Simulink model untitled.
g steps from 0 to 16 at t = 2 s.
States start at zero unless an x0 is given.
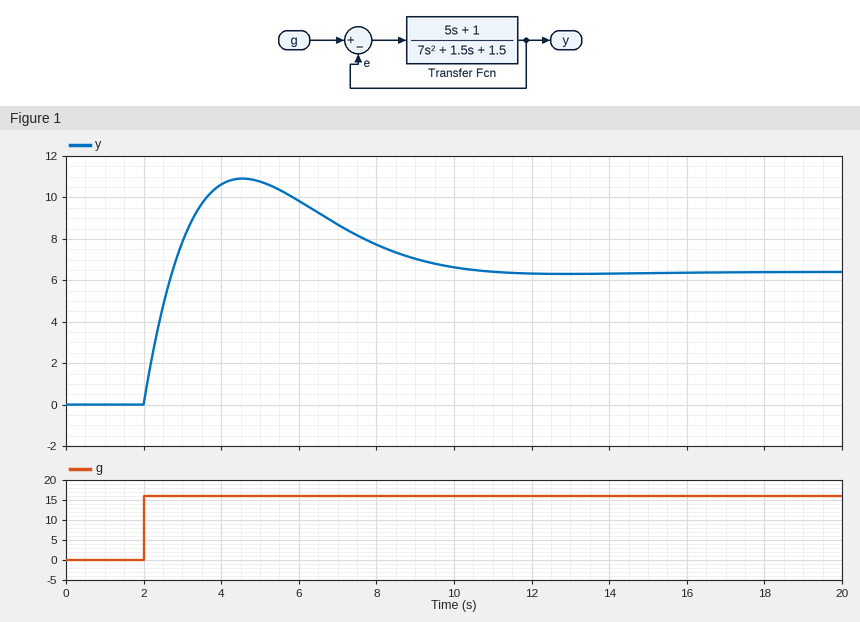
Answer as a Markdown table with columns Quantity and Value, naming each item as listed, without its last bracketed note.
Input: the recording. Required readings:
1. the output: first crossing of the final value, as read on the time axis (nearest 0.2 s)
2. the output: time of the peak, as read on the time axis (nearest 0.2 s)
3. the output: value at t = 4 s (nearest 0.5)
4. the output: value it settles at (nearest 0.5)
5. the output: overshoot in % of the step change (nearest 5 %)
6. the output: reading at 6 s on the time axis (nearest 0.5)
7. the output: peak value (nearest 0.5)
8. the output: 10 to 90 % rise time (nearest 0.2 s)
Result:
| Quantity | Value |
|---|---|
| the output: first crossing of the final value, as read on the time axis | 2.8 s |
| the output: time of the peak, as read on the time axis | 4.6 s |
| the output: value at t = 4 s | 10.5 |
| the output: value it settles at | 6.5 |
| the output: overshoot in % of the step change | 70 % |
| the output: reading at 6 s on the time axis | 10.0 |
| the output: peak value | 11.0 |
| the output: 10 to 90 % rise time | 0.6 s |
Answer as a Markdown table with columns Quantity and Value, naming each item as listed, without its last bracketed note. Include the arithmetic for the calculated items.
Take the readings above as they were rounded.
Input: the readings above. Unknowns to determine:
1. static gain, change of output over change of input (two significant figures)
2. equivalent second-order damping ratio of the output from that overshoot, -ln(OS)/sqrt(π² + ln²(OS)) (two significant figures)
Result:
| Quantity | Value |
|---|---|
| static gain, change of output over change of input | (6.5 - 0) / (16 - 0) = 0.41 |
| equivalent second-order damping ratio of the output from that overshoot, -ln(OS)/sqrt(π² + ln²(OS)) | ln(0.7) = -0.357; 0.357 / sqrt(9.870 + 0.127) = 0.11 |
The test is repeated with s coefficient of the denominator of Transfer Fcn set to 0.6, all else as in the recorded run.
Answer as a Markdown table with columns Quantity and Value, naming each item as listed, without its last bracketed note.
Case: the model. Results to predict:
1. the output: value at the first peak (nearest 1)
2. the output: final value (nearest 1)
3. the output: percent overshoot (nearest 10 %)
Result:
| Quantity | Value |
|---|---|
| the output: value at the first peak | 12 |
| the output: final value | 6 |
| the output: percent overshoot | 90 % |
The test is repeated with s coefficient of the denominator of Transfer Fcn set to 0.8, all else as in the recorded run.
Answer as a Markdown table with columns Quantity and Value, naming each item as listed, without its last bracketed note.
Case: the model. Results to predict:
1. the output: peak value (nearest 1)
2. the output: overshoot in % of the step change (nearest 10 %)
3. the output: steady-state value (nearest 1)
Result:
| Quantity | Value |
|---|---|
| the output: peak value | 12 |
| the output: overshoot in % of the step change | 80 % |
| the output: steady-state value | 6 |
